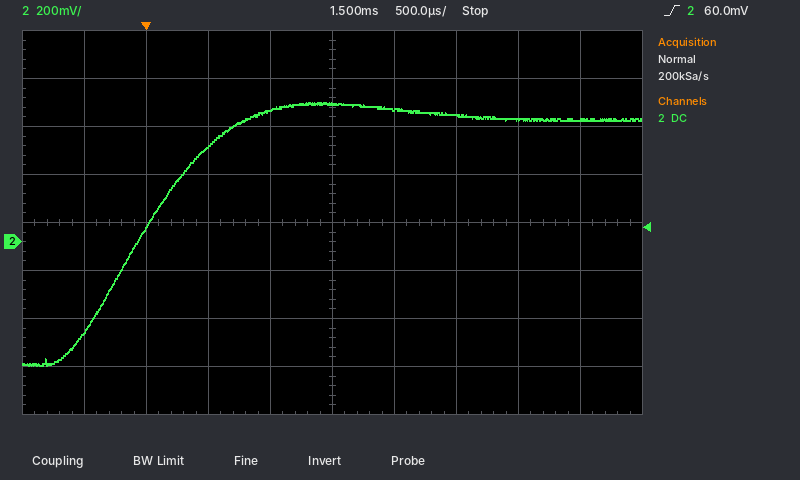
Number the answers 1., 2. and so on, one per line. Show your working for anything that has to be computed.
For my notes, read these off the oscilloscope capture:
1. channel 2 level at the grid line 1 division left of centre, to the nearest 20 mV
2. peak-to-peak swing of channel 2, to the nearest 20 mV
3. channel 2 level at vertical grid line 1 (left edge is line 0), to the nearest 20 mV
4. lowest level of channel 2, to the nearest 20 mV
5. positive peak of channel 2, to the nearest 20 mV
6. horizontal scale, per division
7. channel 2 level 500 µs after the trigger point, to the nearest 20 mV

1. 540 mV
2. 580 mV − (-520 mV) = 1.10 V
3. -380 mV
4. -520 mV
5. 580 mV
6. 500 µs
7. 400 mV
